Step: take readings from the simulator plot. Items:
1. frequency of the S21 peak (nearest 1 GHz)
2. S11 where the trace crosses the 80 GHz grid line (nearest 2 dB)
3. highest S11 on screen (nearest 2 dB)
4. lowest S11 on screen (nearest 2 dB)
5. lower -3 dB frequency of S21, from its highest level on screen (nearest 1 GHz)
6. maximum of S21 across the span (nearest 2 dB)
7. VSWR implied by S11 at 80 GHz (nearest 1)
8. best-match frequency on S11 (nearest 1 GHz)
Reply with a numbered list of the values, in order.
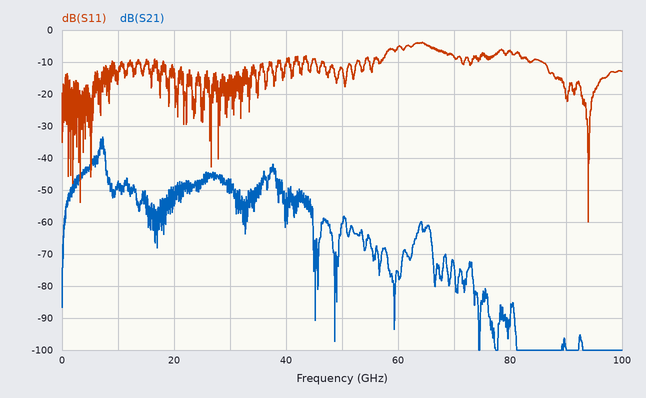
1. 7 GHz
2. -6 dB
3. -4 dB
4. -60 dB
5. 7 GHz
6. -34 dB
7. 3
8. 94 GHz
